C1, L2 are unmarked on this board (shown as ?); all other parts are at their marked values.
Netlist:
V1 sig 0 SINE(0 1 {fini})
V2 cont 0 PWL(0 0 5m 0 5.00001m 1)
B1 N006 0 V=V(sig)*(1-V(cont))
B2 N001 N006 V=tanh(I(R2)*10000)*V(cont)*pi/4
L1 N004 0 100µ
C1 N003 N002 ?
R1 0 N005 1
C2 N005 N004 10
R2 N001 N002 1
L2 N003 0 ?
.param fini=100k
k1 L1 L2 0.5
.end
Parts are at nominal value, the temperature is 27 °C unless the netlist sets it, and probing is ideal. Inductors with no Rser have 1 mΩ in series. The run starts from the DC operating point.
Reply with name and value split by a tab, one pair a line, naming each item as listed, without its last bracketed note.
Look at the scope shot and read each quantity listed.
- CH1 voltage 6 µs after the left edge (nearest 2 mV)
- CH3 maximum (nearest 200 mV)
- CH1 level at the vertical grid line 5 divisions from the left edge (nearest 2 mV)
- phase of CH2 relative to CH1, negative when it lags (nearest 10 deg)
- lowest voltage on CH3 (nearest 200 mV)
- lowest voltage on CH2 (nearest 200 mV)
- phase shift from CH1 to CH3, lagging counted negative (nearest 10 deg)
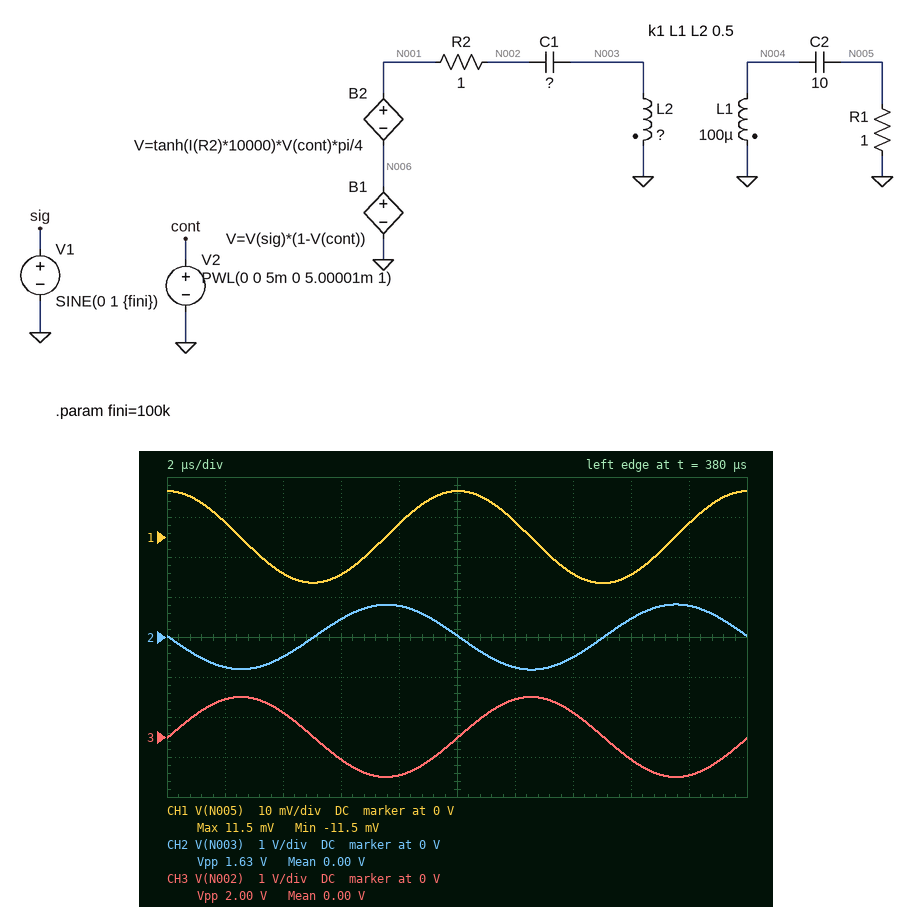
CH1 voltage 6 µs after the left edge	-10 mV
CH3 maximum	1.0 V
CH1 level at the vertical grid line 5 divisions from the left edge	12 mV
phase of CH2 relative to CH1, negative when it lags	90 deg
lowest voltage on CH3	-1.0 V
lowest voltage on CH2	-800 mV
phase shift from CH1 to CH3, lagging counted negative	-90 deg
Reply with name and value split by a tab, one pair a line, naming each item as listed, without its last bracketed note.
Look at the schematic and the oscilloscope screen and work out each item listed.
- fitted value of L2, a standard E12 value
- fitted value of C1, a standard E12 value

fitted value of L2, a standard E12 value	56 µH
fitted value of C1, a standard E12 value	27 nF
